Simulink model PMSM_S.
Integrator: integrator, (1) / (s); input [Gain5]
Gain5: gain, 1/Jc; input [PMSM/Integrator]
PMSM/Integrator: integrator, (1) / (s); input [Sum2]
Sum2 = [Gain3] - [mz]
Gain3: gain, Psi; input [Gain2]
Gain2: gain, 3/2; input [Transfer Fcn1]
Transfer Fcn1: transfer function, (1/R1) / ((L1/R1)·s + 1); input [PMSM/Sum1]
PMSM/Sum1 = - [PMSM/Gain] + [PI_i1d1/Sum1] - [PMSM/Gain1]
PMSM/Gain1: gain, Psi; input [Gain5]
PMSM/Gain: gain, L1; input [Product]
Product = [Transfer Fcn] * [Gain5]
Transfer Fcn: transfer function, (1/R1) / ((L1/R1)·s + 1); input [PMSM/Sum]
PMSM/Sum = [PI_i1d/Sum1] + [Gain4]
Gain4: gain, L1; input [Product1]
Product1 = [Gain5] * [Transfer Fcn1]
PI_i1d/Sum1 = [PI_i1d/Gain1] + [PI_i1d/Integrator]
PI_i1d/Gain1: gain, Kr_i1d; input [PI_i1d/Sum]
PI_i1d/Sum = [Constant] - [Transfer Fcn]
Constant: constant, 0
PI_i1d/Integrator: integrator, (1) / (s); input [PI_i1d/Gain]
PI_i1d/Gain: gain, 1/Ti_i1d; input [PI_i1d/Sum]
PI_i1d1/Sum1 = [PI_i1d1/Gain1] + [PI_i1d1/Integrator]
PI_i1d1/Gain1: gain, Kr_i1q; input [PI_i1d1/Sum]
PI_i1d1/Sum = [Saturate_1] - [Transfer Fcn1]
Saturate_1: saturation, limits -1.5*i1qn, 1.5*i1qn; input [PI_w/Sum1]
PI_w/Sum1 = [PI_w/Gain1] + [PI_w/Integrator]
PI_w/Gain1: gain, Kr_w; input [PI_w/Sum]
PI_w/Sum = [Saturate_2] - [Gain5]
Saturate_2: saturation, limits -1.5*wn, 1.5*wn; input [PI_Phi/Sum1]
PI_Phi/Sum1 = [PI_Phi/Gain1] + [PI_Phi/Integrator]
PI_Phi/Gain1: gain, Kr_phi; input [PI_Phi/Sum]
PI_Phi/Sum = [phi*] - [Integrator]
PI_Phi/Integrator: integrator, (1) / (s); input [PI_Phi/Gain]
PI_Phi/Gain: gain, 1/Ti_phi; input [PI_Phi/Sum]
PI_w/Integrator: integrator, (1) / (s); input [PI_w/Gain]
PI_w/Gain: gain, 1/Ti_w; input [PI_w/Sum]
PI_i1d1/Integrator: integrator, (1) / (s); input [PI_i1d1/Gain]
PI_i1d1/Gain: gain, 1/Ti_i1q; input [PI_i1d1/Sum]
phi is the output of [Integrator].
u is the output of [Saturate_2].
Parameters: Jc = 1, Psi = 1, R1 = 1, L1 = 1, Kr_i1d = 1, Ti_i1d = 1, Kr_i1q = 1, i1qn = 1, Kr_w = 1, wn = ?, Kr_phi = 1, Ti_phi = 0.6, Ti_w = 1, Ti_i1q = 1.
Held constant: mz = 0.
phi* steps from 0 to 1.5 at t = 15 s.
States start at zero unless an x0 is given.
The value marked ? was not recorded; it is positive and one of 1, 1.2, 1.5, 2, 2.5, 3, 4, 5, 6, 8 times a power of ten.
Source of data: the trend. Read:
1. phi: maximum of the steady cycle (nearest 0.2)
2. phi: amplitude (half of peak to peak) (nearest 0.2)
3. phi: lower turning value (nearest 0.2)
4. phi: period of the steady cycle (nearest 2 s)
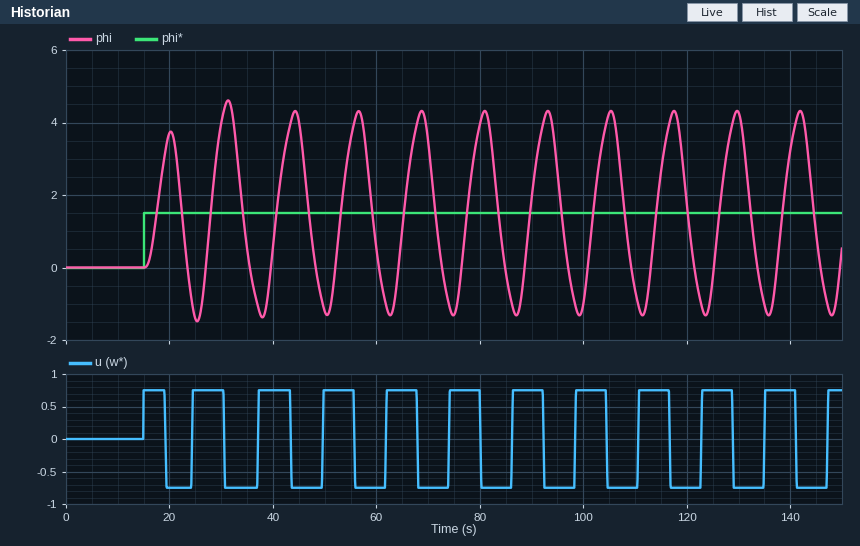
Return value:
4.4
2.8
-1.4
12 s
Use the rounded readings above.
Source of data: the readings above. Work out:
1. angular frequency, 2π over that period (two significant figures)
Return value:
0.52 rad/s
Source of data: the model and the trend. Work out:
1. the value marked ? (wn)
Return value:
0.5
